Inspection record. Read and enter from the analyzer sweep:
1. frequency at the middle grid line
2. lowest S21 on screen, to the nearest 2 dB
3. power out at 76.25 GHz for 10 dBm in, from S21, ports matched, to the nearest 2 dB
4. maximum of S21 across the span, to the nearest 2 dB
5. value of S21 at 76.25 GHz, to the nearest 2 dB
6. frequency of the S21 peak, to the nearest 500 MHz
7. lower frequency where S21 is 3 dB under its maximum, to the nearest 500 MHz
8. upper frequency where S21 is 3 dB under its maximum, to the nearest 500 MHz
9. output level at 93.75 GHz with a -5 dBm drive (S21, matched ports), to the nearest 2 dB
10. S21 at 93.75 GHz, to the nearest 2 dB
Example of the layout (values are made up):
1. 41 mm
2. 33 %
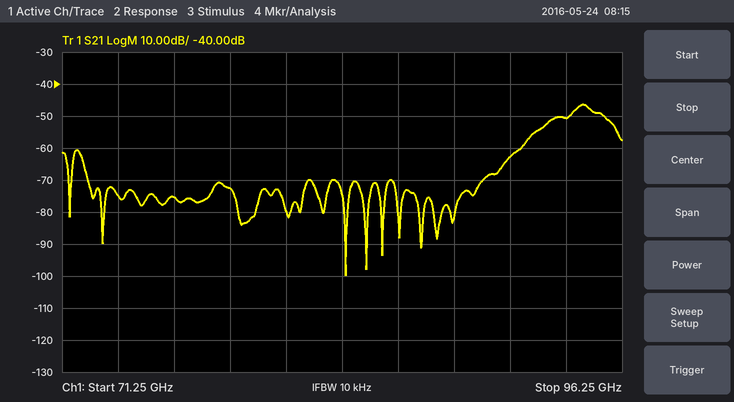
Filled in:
1. 83.75 GHz
2. -100 dB
3. -66 dBm
4. -46 dB
5. -76 dB
6. 94.5 GHz
7. 94.0 GHz
8. 95.5 GHz
9. -56 dBm
10. -50 dB
